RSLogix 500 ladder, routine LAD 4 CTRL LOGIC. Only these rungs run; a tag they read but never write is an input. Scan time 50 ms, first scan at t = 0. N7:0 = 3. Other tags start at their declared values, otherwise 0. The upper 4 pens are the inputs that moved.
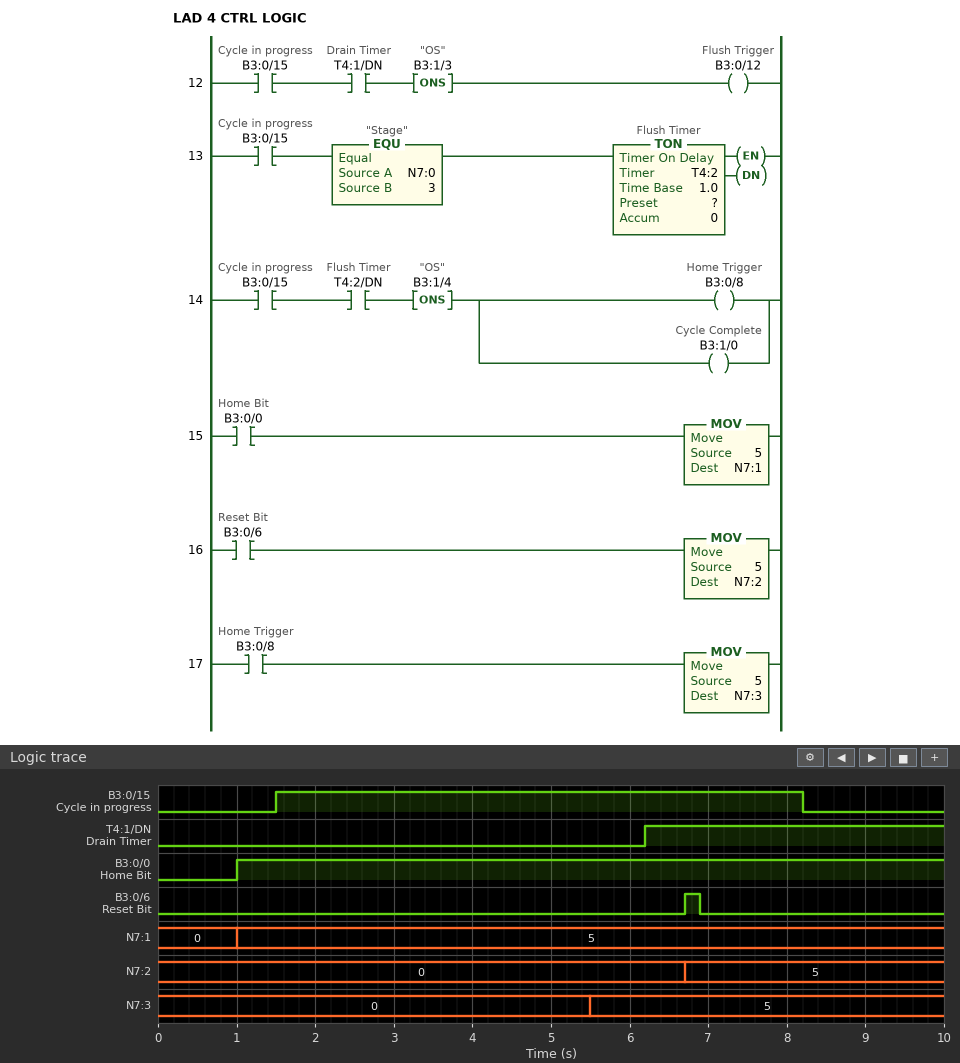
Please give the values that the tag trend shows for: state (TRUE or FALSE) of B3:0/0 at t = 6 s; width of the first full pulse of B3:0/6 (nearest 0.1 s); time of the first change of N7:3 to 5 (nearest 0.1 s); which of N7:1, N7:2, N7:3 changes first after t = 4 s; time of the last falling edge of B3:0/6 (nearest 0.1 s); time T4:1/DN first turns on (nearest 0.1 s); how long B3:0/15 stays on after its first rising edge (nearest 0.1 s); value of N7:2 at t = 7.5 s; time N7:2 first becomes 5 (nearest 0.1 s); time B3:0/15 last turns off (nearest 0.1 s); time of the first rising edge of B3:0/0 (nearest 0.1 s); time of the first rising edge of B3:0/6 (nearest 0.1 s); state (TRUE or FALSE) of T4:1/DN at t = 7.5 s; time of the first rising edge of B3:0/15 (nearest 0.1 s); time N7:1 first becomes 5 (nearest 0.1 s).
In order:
TRUE
0.2 s
5.5 s
N7:3
6.9 s
6.2 s
6.7 s
5
6.7 s
8.2 s
1.0 s
6.7 s
TRUE
1.5 s
1.0 s
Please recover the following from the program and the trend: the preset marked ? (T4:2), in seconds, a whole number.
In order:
4 s
